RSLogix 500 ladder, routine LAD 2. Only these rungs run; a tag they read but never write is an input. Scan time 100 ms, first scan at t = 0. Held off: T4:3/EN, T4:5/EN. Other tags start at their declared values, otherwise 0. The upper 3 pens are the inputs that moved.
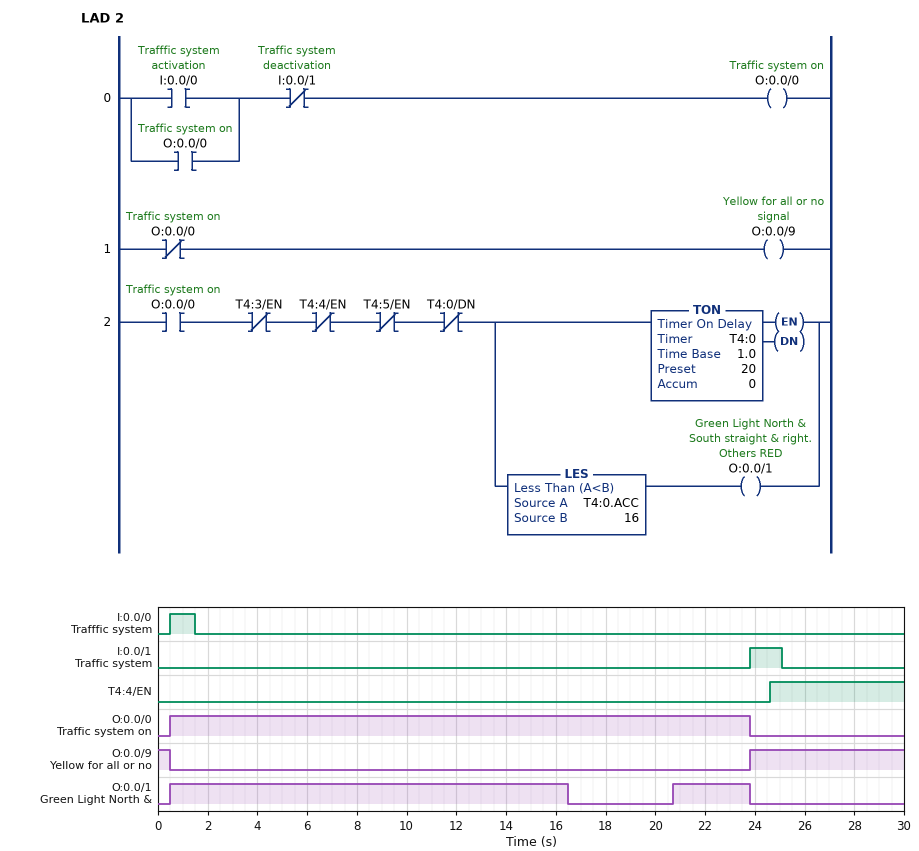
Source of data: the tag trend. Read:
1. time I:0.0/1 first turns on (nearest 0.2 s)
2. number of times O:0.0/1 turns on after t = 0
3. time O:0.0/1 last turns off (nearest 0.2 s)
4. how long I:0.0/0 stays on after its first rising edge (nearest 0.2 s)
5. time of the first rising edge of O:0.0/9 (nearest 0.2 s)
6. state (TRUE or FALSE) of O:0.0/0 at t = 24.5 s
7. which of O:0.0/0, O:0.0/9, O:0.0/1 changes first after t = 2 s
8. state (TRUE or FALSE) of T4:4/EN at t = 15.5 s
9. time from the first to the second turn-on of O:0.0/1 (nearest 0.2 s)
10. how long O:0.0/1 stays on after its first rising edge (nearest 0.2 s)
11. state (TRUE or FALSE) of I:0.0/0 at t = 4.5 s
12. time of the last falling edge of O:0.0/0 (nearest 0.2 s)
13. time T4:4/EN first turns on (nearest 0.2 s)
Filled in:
23.8 s
2
23.8 s
1.0 s
23.8 s
FALSE
O:0.0/1
FALSE
20.2 s
16.0 s
FALSE
23.8 s
24.6 s
